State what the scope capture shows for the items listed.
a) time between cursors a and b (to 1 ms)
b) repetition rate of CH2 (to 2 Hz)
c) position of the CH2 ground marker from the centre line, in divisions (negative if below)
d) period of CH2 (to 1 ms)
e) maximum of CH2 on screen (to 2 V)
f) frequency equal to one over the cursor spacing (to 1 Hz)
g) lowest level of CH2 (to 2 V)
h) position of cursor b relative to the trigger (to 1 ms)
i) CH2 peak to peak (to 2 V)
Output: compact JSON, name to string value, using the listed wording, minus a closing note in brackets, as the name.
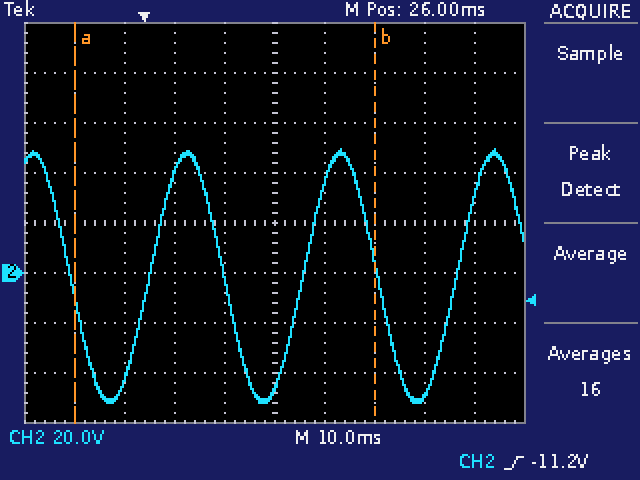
{"time between cursors a and b": "60 ms", "repetition rate of CH2": "32 Hz", "position of the CH2 ground marker from the centre line, in divisions": "-1.0 div", "period of CH2": "31 ms", "maximum of CH2 on screen": "50 V", "frequency equal to one over the cursor spacing": "17 Hz", "lowest level of CH2": "-52 V", "position of cursor b relative to the trigger": "+46 ms", "CH2 peak to peak": "102 V"}
